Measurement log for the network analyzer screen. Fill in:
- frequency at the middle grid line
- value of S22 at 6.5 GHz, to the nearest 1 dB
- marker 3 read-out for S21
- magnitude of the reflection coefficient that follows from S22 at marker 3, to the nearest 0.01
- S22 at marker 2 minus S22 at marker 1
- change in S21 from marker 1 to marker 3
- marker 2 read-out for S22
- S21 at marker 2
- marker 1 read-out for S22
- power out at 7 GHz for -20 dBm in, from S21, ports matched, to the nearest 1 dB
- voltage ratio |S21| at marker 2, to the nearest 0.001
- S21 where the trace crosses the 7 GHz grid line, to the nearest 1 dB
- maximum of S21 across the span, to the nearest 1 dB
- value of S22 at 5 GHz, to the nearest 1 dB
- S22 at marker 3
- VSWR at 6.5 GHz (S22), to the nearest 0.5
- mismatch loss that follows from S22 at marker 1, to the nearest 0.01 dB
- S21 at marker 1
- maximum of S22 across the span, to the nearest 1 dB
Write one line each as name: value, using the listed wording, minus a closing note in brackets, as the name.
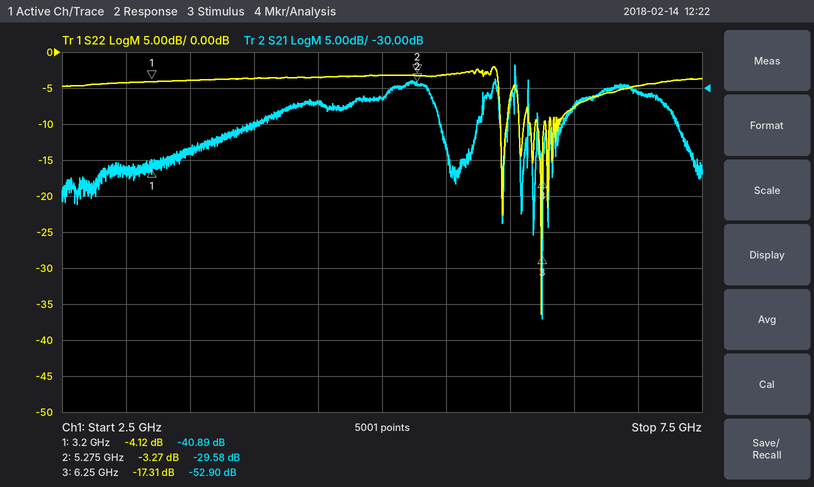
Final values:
frequency at the middle grid line: 5 GHz
value of S22 at 6.5 GHz, to the nearest 1 dB: -8 dB
marker 3 read-out for S21: -52.90 dB
magnitude of the reflection coefficient that follows from S22 at marker 3, to the nearest 0.01: 0.14
S22 at marker 2 minus S22 at marker 1: 0.85 dB
change in S21 from marker 1 to marker 3: -12.01 dB
marker 2 read-out for S22: -3.27 dB
S21 at marker 2: -29.58 dB
marker 1 read-out for S22: -4.12 dB
power out at 7 GHz for -20 dBm in, from S21, ports matched, to the nearest 1 dB: -51 dBm
voltage ratio |S21| at marker 2, to the nearest 0.001: 0.033
S21 where the trace crosses the 7 GHz grid line, to the nearest 1 dB: -31 dB
maximum of S21 across the span, to the nearest 1 dB: -27 dB
value of S22 at 5 GHz, to the nearest 1 dB: -3 dB
S22 at marker 3: -17.31 dB
VSWR at 6.5 GHz (S22), to the nearest 0.5: 2.5
mismatch loss that follows from S22 at marker 1, to the nearest 0.01 dB: 2.13 dB
S21 at marker 1: -40.89 dB
maximum of S22 across the span, to the nearest 1 dB: -2 dB
